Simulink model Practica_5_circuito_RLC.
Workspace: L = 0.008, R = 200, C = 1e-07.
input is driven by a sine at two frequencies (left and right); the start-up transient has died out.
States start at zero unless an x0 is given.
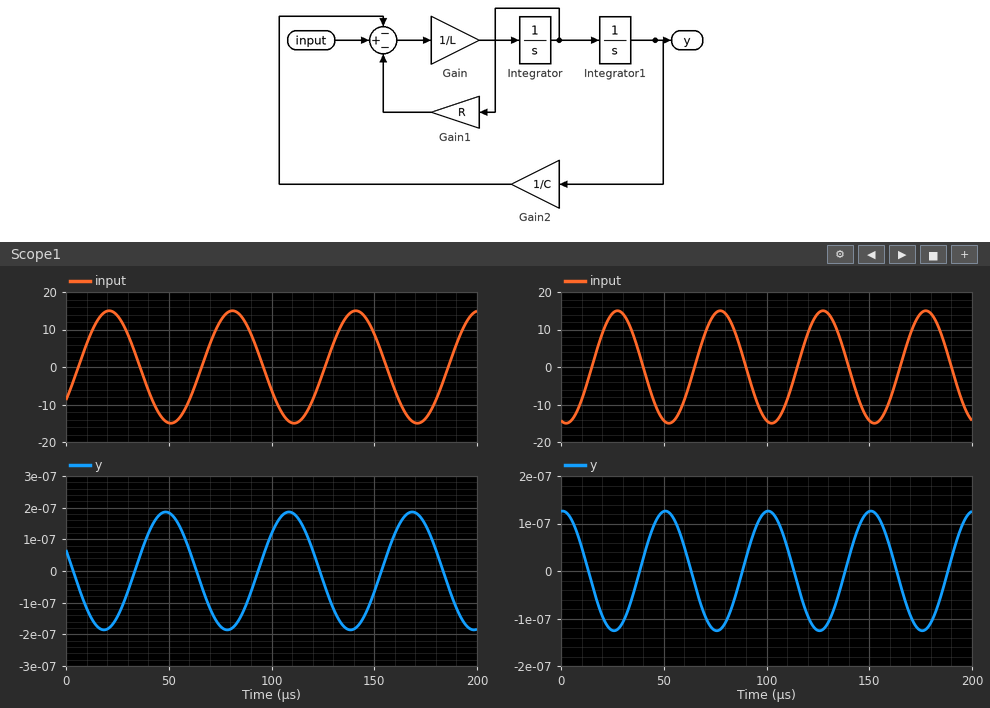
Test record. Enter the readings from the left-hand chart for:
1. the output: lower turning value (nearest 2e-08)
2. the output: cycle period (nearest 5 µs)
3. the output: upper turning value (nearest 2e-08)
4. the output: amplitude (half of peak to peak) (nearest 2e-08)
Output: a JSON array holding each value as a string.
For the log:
["-0.00000018", "60 µs", "0.00000018", "0.00000018"]
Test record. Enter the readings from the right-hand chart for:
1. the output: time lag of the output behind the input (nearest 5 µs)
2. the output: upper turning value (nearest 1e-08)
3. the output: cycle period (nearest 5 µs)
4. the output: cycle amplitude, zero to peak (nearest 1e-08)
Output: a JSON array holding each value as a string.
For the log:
["25 µs", "0.00000013", "50 µs", "0.00000013"]
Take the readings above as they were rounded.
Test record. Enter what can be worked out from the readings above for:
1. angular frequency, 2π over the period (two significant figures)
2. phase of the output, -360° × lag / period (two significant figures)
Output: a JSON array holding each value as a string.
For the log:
["0.13 rad/µs", "-180°"]
